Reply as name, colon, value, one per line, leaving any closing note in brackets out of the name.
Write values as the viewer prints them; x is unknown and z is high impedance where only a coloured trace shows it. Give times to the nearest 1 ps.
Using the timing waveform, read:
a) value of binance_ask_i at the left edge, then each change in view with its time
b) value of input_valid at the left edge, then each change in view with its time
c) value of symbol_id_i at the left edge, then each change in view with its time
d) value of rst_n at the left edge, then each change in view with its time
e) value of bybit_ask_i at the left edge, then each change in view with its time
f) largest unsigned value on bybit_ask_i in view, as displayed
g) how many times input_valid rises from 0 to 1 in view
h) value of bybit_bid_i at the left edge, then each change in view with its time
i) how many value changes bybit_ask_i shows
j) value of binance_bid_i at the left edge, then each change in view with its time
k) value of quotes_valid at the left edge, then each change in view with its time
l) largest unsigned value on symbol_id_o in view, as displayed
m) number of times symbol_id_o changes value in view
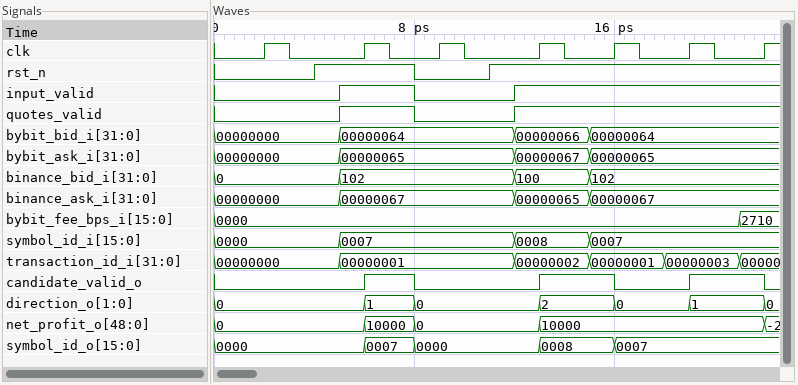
value of binance_ask_i at the left edge, then each change in view with its time: 00000000, 00000067 at 5 ps, 00000065 at 12 ps, 00000067 at 15 ps
value of input_valid at the left edge, then each change in view with its time: 0, 1 at 5 ps, 0 at 8 ps, 1 at 12 ps
value of symbol_id_i at the left edge, then each change in view with its time: 0000, 0007 at 5 ps, 0008 at 12 ps, 0007 at 15 ps
value of rst_n at the left edge, then each change in view with its time: 0, 1 at 4 ps, 0 at 8 ps, 1 at 11 ps
value of bybit_ask_i at the left edge, then each change in view with its time: 00000000, 00000065 at 5 ps, 00000067 at 12 ps, 00000065 at 15 ps
largest unsigned value on bybit_ask_i in view, as displayed: 00000067
how many times input_valid rises from 0 to 1 in view: 2
value of bybit_bid_i at the left edge, then each change in view with its time: 00000000, 00000064 at 5 ps, 00000066 at 12 ps, 00000064 at 15 ps
how many value changes bybit_ask_i shows: 3
value of binance_bid_i at the left edge, then each change in view with its time: 0, 102 at 5 ps, 100 at 12 ps, 102 at 15 ps
value of quotes_valid at the left edge, then each change in view with its time: 0, 1 at 5 ps, 0 at 8 ps, 1 at 12 ps
largest unsigned value on symbol_id_o in view, as displayed: 0008
number of times symbol_id_o changes value in view: 4
